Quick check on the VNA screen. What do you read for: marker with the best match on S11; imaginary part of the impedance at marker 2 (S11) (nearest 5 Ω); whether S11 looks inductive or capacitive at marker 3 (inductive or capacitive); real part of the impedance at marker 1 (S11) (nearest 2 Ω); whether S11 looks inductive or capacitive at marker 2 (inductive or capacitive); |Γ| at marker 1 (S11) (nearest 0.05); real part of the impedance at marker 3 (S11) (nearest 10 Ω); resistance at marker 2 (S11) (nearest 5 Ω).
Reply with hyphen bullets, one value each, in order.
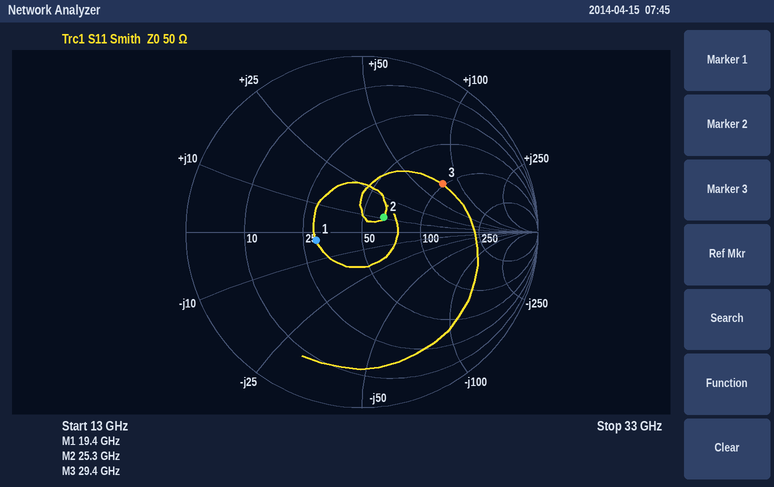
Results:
- marker 2
- +10 Ω
- inductive
- 30 Ω
- inductive
- 0.25
- 100 Ω
- 65 Ω
